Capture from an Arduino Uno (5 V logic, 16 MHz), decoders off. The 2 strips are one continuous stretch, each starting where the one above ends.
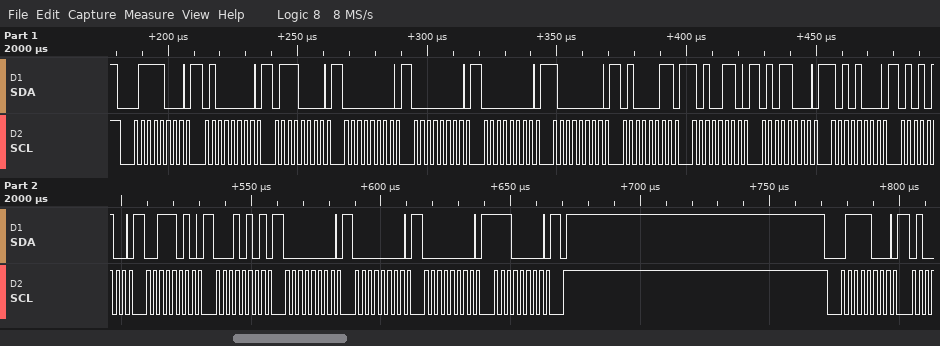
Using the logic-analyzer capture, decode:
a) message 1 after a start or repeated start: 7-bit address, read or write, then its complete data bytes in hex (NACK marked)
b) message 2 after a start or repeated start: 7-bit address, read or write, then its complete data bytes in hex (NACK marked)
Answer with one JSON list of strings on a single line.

["0x3C write: 40 70 00 00 00 80 43 A6 58 A8 54 3A 15 00 00 00 E0", "0x3C write"]
